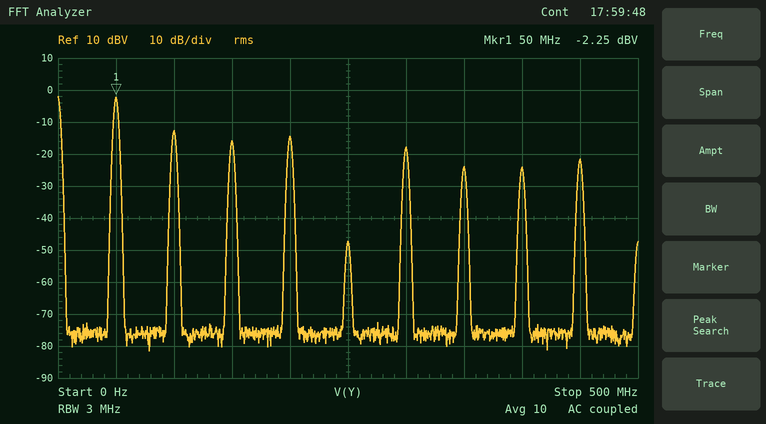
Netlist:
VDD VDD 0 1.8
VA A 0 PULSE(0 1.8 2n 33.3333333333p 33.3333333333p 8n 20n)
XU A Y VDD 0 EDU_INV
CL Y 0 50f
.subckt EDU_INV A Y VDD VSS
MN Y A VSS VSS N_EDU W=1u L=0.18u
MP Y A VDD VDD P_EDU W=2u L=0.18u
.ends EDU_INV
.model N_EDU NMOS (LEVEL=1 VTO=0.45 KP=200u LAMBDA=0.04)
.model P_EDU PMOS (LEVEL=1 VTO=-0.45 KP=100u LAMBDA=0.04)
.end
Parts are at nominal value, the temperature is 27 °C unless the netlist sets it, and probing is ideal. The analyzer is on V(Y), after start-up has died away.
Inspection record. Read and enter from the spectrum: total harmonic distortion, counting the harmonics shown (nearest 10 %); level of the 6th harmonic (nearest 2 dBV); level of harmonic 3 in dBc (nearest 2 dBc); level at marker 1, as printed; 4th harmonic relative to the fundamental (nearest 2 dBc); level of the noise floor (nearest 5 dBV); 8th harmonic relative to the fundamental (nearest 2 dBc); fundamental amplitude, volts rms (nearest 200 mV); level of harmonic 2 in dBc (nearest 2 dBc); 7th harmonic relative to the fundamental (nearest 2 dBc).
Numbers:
50 %
-18 dBV
-14 dBc
-2.25 dBV
-12 dBc
-75 dBV
-22 dBc
800 mV
-10 dBc
-22 dBc
